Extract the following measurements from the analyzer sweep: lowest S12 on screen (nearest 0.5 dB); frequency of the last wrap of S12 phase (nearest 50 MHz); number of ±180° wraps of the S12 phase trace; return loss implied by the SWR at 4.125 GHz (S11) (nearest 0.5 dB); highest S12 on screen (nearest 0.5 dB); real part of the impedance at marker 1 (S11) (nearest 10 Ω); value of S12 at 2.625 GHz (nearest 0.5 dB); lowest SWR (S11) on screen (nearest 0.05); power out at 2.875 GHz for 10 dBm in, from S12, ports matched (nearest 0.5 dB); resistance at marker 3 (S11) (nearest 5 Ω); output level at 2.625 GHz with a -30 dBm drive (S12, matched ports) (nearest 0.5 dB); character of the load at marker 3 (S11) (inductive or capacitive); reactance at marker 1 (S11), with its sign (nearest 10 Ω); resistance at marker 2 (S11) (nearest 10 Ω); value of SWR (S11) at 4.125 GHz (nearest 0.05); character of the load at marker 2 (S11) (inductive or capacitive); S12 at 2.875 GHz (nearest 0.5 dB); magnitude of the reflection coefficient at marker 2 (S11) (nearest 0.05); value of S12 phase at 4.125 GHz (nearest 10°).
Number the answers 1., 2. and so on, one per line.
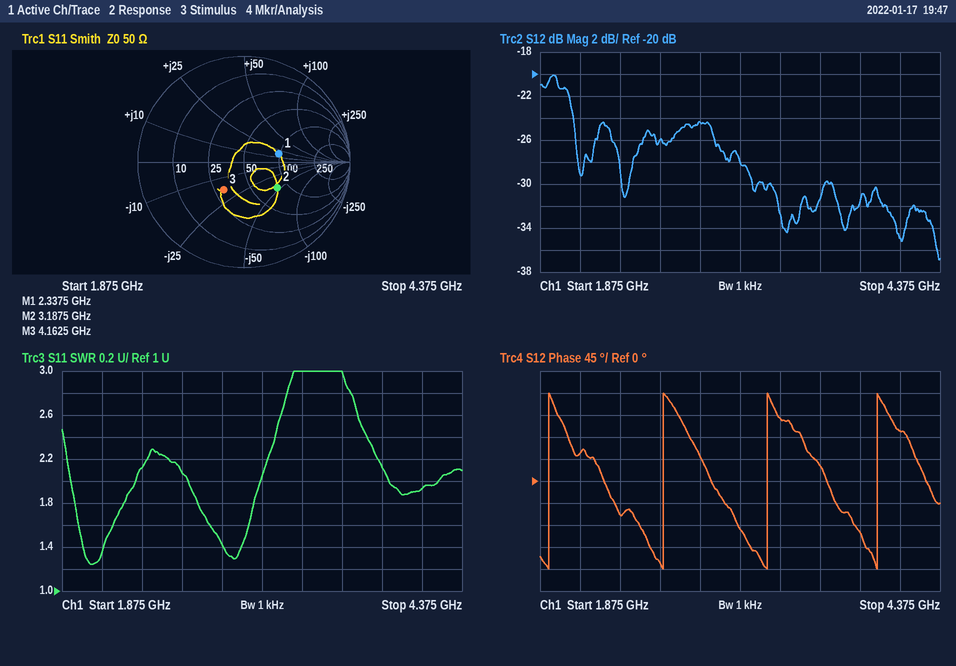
1. -37.0 dB
2. 4.00 GHz
3. 4
4. 10.0 dB
5. -20.0 dB
6. 100 Ω
7. -26.0 dB
8. 1.25
9. -14.5 dBm
10. 30 Ω
11. -56.0 dBm
12. capacitive
13. +20 Ω
14. 80 Ω
15. 1.95
16. capacitive
17. -24.5 dB
18. 0.40
19. 100°
